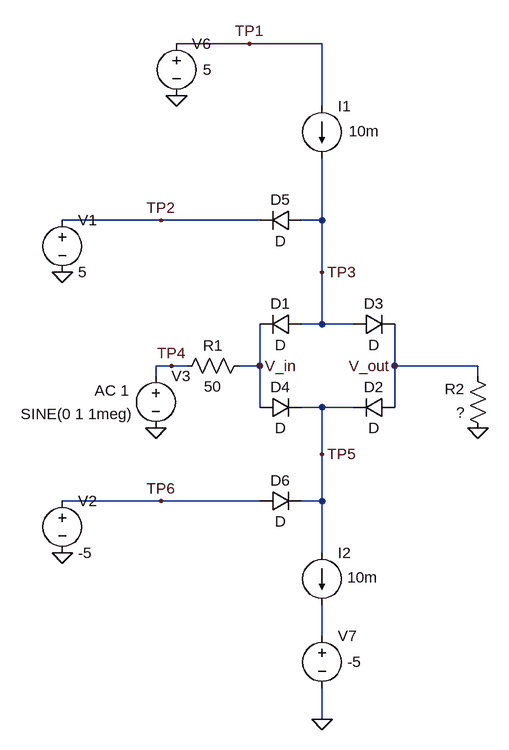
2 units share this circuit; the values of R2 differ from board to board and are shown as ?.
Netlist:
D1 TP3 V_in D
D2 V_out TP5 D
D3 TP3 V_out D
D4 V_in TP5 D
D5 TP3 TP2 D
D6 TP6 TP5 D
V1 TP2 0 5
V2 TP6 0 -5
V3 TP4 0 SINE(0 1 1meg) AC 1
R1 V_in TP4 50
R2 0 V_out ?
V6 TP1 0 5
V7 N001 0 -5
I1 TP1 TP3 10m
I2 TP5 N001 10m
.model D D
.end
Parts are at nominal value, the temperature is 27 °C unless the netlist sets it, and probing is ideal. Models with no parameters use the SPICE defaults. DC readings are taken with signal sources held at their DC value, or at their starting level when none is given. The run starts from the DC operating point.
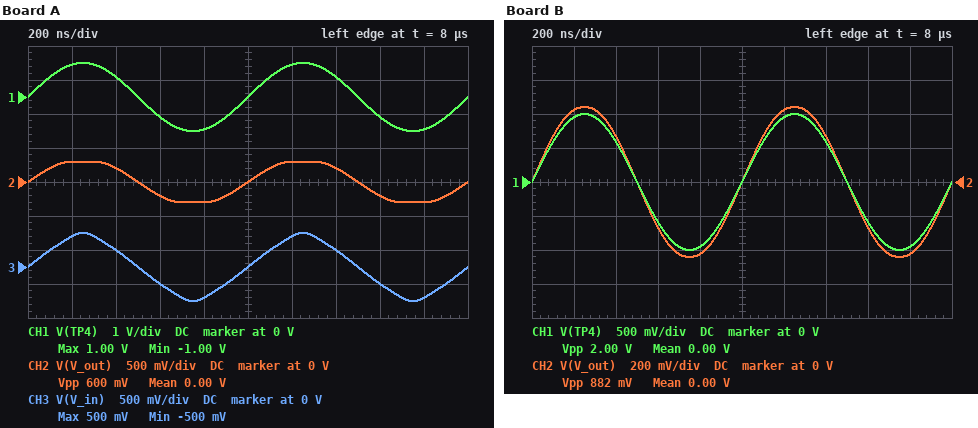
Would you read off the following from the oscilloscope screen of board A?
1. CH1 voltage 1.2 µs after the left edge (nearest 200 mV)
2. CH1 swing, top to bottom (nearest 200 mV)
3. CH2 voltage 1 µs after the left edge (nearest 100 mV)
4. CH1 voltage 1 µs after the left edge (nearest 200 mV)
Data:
1.0 V
2.0 V
0 V
0 V
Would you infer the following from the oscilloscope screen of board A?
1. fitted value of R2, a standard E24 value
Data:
30 Ω
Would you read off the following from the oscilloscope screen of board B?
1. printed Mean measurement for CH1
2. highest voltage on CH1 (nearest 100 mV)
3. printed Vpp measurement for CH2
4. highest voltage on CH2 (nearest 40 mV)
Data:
0.00 V
1.0 V
882 mV
440 mV
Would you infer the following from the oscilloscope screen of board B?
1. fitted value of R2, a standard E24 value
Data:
47 Ω
